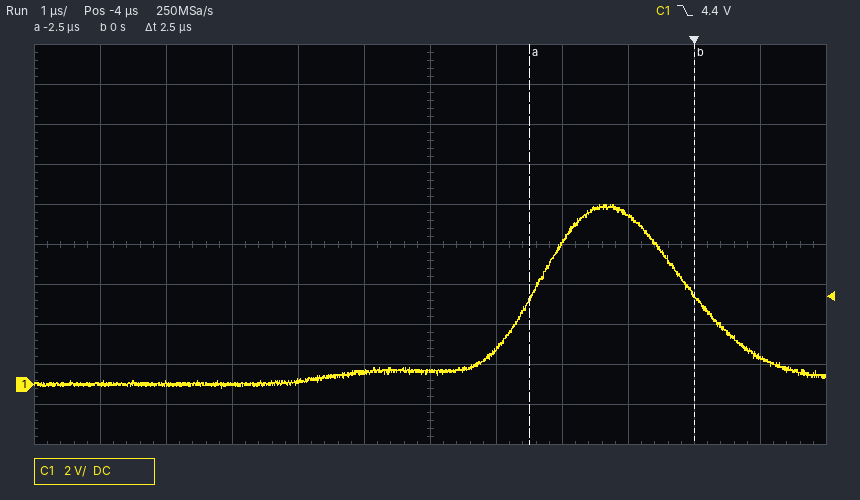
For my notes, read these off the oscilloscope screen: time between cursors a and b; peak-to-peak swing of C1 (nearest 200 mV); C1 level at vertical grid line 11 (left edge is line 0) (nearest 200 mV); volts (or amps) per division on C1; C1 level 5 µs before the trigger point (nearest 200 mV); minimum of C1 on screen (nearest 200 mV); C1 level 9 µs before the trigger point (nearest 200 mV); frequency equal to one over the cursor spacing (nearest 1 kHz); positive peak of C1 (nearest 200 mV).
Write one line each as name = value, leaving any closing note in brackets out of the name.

time between cursors a and b = 2.5 µs
peak-to-peak swing of C1 = 9.2 V
C1 level at vertical grid line 11 (left edge is line 0) = 1.4 V
volts (or amps) per division on C1 = 2 V
C1 level 5 µs before the trigger point = 600 mV
minimum of C1 on screen = -200 mV
C1 level 9 µs before the trigger point = 0.0 V
frequency equal to one over the cursor spacing = 400 kHz
positive peak of C1 = 9.0 V
